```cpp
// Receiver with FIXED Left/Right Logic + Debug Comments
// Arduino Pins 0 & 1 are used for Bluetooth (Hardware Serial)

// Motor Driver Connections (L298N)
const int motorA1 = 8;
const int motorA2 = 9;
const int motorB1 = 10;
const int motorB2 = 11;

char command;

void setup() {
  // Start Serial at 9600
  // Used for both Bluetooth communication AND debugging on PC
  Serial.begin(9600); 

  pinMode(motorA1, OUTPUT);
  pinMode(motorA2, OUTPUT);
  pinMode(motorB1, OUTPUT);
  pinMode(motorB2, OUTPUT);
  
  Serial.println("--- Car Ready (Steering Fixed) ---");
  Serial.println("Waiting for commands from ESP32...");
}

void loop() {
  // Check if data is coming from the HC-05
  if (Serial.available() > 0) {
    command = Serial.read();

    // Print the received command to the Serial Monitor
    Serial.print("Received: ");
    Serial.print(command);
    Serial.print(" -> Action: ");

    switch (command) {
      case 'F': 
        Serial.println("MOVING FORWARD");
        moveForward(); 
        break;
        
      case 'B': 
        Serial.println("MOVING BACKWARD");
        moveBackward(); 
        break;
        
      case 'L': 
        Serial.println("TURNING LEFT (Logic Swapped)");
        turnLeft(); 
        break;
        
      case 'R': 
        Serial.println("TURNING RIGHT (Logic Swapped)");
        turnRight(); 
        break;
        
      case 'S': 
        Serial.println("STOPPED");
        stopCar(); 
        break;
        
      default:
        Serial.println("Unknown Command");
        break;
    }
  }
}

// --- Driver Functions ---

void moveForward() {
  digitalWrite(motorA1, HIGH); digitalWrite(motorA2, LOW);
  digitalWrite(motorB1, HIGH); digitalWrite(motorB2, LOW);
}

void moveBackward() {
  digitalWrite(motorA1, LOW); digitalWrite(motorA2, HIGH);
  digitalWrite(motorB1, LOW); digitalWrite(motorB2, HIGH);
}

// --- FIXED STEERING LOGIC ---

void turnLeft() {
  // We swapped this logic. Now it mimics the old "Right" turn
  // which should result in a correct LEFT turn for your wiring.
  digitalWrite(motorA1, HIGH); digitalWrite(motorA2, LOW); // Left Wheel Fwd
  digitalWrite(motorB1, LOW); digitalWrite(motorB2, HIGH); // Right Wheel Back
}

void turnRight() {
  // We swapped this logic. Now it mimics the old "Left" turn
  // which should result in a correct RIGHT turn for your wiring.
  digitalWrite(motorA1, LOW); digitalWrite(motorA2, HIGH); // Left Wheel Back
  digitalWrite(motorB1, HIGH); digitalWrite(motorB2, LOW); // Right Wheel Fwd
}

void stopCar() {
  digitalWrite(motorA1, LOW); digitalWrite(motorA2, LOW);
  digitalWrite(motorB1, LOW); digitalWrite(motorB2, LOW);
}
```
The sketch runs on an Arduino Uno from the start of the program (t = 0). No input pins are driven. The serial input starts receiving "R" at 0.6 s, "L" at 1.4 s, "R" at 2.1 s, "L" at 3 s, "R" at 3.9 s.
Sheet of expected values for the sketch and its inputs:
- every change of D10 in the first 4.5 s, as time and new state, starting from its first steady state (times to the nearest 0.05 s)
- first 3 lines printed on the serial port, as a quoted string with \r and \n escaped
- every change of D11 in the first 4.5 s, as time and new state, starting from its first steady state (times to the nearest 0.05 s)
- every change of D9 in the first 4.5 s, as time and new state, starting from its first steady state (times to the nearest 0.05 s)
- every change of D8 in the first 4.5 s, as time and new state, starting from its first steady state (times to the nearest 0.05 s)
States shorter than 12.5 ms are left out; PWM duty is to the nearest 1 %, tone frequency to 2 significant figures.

0 s low; 0.6 s high; 1.4 s low; 2.1 s high; 3 s low; 3.9 s high
"--- Car Ready (Steering Fixed) ---\r\nWaiting for commands from ESP32...\r\nReceived: R -> Action: TURNING RIGHT (Logic Swapped)\r\n"
0 s low; 1.4 s high; 2.1 s low; 3 s high; 3.9 s low
0 s low; 0.6 s high; 1.4 s low; 2.1 s high; 3 s low; 3.9 s high
0 s low; 1.4 s high; 2.1 s low; 3 s high; 3.9 s low
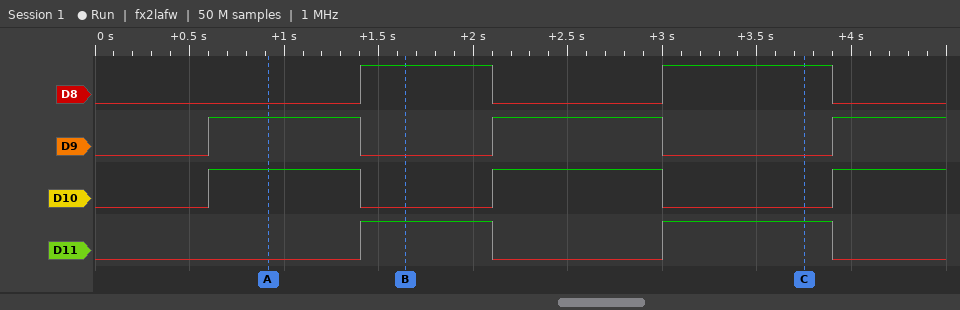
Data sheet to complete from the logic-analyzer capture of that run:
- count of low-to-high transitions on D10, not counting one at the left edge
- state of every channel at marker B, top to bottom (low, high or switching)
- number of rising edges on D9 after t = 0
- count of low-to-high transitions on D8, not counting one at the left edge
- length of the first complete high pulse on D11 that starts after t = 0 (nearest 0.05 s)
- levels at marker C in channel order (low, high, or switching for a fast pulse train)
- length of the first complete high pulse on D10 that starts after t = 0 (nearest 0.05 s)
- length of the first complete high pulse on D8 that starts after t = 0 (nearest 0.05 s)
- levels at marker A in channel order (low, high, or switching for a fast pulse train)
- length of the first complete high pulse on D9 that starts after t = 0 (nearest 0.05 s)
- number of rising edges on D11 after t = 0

3
D8 high, D9 low, D10 low, D11 high
3
2
0.70 s
D8 high, D9 low, D10 low, D11 high
0.80 s
0.70 s
D8 low, D9 high, D10 high, D11 low
0.80 s
2
